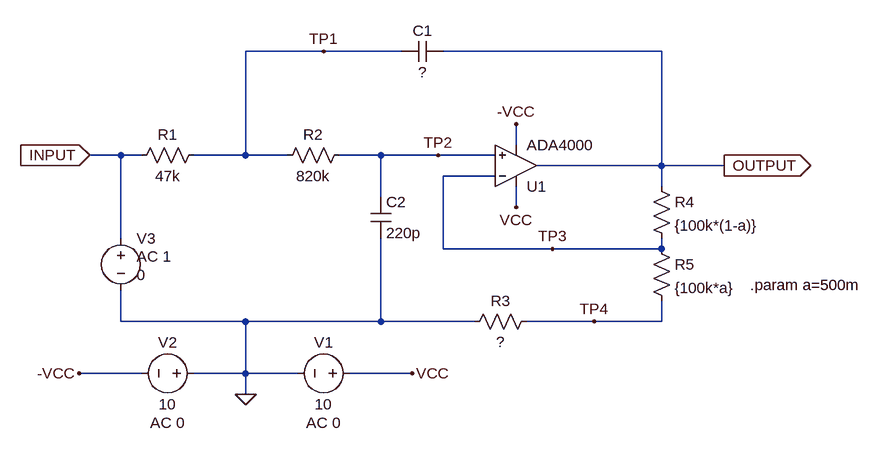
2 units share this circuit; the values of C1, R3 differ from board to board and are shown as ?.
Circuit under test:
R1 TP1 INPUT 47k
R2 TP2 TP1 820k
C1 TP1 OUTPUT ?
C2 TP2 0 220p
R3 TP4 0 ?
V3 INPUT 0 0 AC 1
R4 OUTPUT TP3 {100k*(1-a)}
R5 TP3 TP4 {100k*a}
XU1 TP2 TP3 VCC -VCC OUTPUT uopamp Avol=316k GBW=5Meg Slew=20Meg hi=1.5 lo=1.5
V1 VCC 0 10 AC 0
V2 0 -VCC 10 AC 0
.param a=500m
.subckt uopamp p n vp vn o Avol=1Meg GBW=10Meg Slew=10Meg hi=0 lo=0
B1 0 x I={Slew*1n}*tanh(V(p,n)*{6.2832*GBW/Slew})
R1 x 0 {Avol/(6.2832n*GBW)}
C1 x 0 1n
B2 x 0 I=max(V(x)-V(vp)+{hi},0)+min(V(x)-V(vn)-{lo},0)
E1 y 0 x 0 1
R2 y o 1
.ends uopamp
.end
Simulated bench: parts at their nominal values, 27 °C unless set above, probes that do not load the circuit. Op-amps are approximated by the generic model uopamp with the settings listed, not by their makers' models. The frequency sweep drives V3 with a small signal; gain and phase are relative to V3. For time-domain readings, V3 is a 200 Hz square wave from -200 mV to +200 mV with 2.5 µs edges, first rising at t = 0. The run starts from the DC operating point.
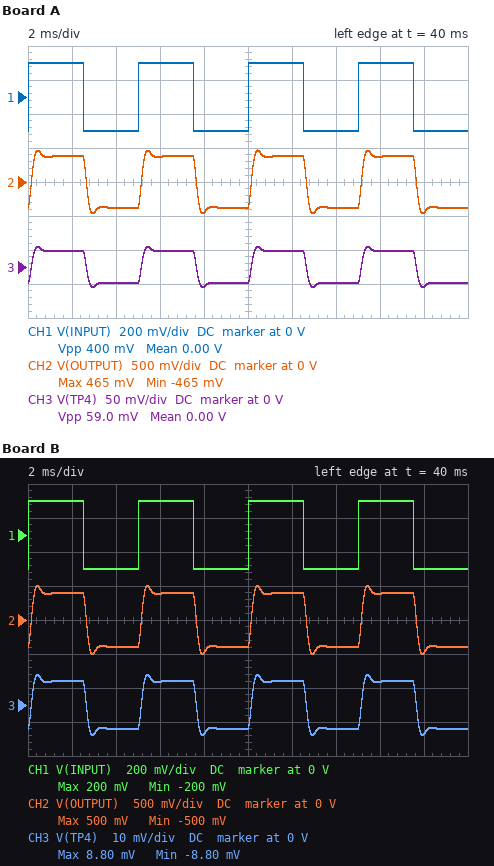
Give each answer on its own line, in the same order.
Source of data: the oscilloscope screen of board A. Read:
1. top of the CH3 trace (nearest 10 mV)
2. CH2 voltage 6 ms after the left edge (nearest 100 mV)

30 mV
400 mV
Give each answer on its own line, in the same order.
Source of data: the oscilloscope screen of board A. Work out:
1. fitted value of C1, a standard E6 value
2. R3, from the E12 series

1.5 nF
6.8 kΩ
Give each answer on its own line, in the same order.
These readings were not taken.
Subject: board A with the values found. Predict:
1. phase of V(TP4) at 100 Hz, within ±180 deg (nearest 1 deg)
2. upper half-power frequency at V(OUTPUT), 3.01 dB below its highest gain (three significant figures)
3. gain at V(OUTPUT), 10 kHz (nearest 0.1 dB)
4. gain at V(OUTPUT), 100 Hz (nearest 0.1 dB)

-5 deg
1.60 kHz
-28.5 dB
5.5 dB
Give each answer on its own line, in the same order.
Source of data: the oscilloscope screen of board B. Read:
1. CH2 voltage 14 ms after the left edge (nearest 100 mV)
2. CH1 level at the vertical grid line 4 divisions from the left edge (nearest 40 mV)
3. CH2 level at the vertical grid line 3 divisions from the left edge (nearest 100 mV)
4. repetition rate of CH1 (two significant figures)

-400 mV
-200 mV
400 mV
200 Hz
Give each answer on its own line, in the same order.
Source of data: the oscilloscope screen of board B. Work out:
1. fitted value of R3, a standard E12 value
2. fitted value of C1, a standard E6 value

1.8 kΩ
1.5 nF
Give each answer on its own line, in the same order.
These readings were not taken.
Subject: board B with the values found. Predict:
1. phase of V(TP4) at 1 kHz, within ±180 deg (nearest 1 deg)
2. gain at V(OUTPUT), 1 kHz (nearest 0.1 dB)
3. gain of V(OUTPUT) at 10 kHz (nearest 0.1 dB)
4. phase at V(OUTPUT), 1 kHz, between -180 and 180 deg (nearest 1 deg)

-57 deg
6.6 dB
-28.1 dB
-57 deg
